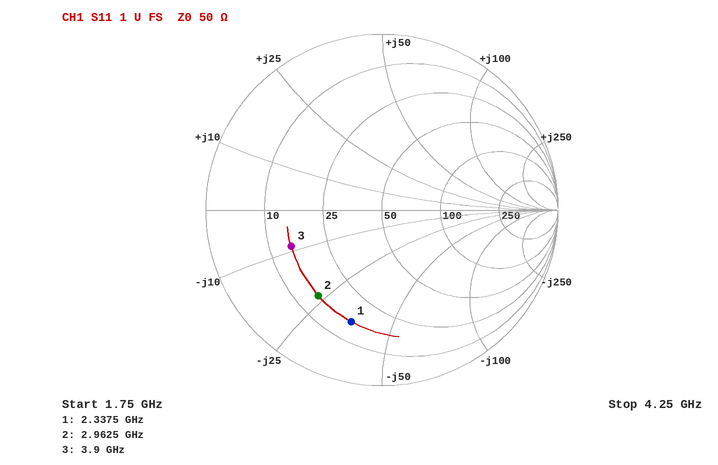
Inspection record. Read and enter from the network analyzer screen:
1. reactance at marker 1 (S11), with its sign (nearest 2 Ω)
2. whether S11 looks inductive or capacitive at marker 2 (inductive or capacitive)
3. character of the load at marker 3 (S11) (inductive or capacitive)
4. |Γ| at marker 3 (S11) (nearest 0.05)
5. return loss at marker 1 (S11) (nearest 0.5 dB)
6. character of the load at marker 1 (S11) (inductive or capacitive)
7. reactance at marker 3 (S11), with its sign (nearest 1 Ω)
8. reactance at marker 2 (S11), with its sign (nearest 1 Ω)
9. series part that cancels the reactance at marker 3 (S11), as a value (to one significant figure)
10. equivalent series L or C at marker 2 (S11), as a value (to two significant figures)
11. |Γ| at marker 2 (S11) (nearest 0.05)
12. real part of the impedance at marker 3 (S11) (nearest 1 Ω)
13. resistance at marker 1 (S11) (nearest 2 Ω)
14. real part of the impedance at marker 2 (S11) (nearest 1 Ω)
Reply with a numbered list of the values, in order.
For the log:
1. -36 Ω
2. capacitive
3. capacitive
4. 0.55
5. 3.5 dB
6. capacitive
7. -9 Ω
8. -23 Ω
9. 400 pH
10. 2.3 pF
11. 0.60
12. 15 Ω
13. 16 Ω
14. 15 Ω
